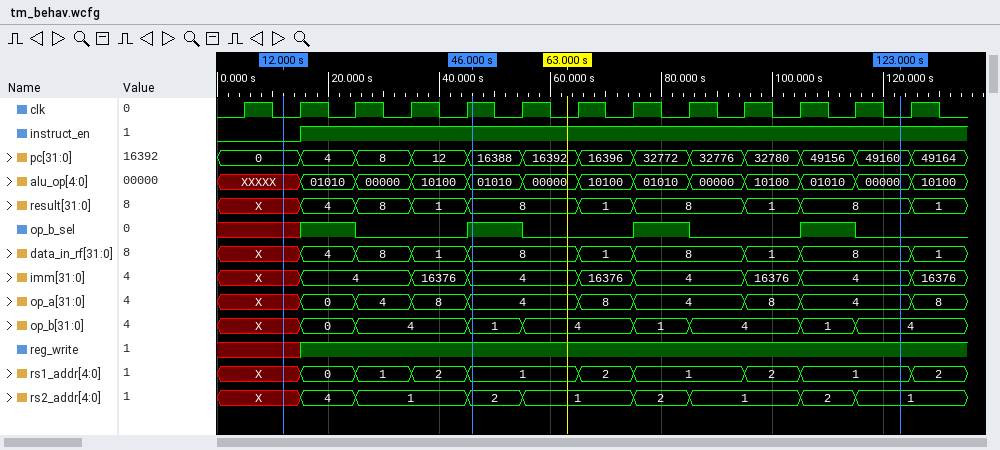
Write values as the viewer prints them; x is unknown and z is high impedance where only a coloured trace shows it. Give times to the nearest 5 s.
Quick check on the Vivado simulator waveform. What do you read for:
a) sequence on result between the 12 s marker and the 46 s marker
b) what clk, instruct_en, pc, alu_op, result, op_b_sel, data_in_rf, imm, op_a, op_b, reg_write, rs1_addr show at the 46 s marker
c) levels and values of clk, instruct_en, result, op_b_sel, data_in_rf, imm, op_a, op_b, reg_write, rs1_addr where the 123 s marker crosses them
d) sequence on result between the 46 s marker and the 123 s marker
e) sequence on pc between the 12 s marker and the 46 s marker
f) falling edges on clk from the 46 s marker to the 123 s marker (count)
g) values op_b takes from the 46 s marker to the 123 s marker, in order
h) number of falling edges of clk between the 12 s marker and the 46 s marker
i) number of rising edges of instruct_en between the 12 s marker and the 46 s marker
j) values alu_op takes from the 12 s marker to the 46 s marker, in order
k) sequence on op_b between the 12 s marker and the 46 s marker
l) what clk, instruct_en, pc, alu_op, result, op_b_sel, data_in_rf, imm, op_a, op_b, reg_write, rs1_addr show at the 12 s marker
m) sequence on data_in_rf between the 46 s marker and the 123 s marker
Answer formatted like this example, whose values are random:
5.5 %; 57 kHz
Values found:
X, 4, 8, 1, 8; clk=1, instruct_en=1, pc=16388, alu_op=01010, result=8, op_b_sel=1, data_in_rf=8, imm=4, op_a=4, op_b=1, reg_write=1, rs1_addr=1; clk=0, instruct_en=1, result=8, op_b_sel=0, data_in_rf=8, imm=4, op_a=4, op_b=4, reg_write=1, rs1_addr=1; 8, 1, 8, 1, 8; 0, 4, 8, 12, 16388; 8; 1, 4, 1, 4, 1, 4; 3; 1; XXXXX, 01010, 00000, 10100, 01010; X, 0, 4, 1; clk=0, instruct_en=0, pc=0, alu_op=XXXXX, result=X, op_b_sel=x, data_in_rf=X, imm=X, op_a=X, op_b=X, reg_write=x, rs1_addr=X; 8, 1, 8, 1, 8
